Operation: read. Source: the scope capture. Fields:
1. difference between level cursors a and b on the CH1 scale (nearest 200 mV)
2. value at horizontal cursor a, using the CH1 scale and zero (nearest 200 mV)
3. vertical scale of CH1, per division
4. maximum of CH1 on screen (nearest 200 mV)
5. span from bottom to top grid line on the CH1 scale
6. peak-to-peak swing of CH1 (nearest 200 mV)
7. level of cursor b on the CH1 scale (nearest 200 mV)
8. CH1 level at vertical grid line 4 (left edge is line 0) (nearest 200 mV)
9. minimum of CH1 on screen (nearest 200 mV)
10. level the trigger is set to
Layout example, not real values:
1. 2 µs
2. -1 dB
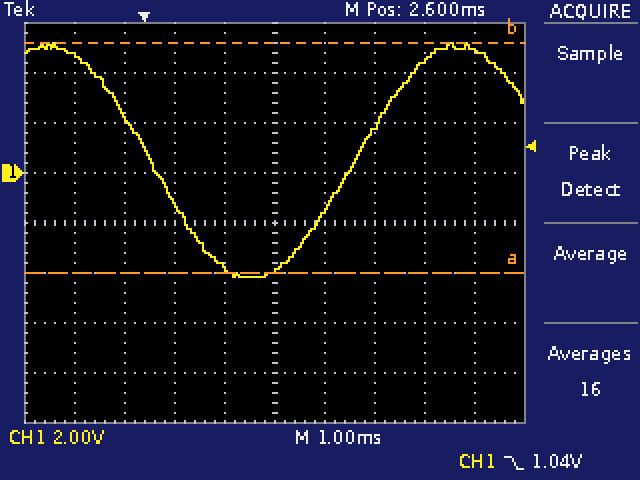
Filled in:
1. 9.2 V
2. -4.0 V
3. 2 V
4. 5.2 V
5. 16 V
6. 9.4 V
7. 5.2 V
8. -3.8 V
9. -4.2 V
10. 1.04 V
